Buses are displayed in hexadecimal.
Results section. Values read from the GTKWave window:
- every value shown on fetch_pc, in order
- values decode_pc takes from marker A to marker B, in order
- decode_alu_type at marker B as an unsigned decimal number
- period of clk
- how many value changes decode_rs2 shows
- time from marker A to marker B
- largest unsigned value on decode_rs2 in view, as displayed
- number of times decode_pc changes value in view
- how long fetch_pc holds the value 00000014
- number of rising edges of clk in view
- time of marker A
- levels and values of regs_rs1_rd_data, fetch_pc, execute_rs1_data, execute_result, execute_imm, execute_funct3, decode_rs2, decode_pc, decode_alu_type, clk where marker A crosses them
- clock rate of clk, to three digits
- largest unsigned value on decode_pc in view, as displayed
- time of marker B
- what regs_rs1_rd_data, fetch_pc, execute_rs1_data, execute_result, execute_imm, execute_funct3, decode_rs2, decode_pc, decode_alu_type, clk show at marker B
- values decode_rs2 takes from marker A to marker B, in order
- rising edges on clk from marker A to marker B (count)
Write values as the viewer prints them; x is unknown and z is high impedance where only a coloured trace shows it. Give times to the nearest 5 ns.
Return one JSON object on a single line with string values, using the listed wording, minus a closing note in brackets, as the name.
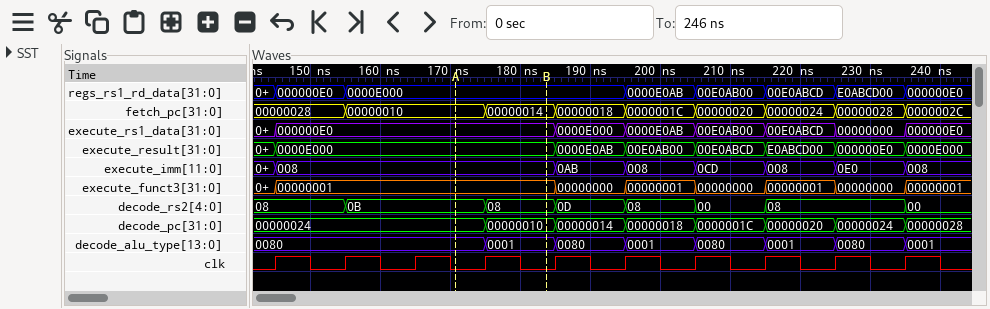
{"every value shown on fetch_pc, in order": "00000028, 00000010, 00000014, 00000018, 0000001C, 00000020, 00000024, 00000028, 0000002C", "values decode_pc takes from marker A to marker B, in order": "00000024, 00000010", "decode_alu_type at marker B as an unsigned decimal number": "1", "period of clk": "10 ns", "how many value changes decode_rs2 shows": "7", "time from marker A to marker B": "15 ns", "largest unsigned value on decode_rs2 in view, as displayed": "0D", "number of times decode_pc changes value in view": "7", "how long fetch_pc holds the value 00000014": "10 ns", "number of rising edges of clk in view": "10", "time of marker A": "170 ns", "levels and values of regs_rs1_rd_data, fetch_pc, execute_rs1_data, execute_result, execute_imm, execute_funct3, decode_rs2, decode_pc, decode_alu_type, clk where marker A crosses them": "regs_rs1_rd_data=0000E000, fetch_pc=00000010, execute_rs1_data=000000E0, execute_result=0000E000, execute_imm=008, execute_funct3=00000001, decode_rs2=0B, decode_pc=00000024, decode_alu_type=0080, clk=0", "clock rate of clk, to three digits": "100 MHz", "largest unsigned value on decode_pc in view, as displayed": "00000028", "time of marker B": "185 ns", "what regs_rs1_rd_data, fetch_pc, execute_rs1_data, execute_result, execute_imm, execute_funct3, decode_rs2, decode_pc, decode_alu_type, clk show at marker B": "regs_rs1_rd_data=0000E000, fetch_pc=00000014, execute_rs1_data=000000E0, execute_result=0000E000, execute_imm=008, execute_funct3=00000001, decode_rs2=08, decode_pc=00000010, decode_alu_type=0001, clk=0", "values decode_rs2 takes from marker A to marker B, in order": "0B, 08", "rising edges on clk from marker A to marker B": "1"}
